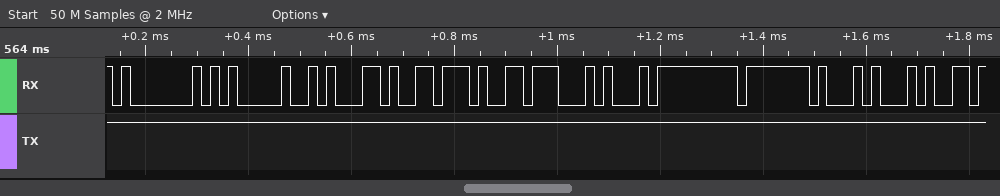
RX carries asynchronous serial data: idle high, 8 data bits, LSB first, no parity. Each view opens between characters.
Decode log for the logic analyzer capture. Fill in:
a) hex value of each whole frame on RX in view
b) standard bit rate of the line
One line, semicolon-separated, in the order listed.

01, 05, 8A, D9, D9, 14, FF, 7F, 14; 57600 baud
